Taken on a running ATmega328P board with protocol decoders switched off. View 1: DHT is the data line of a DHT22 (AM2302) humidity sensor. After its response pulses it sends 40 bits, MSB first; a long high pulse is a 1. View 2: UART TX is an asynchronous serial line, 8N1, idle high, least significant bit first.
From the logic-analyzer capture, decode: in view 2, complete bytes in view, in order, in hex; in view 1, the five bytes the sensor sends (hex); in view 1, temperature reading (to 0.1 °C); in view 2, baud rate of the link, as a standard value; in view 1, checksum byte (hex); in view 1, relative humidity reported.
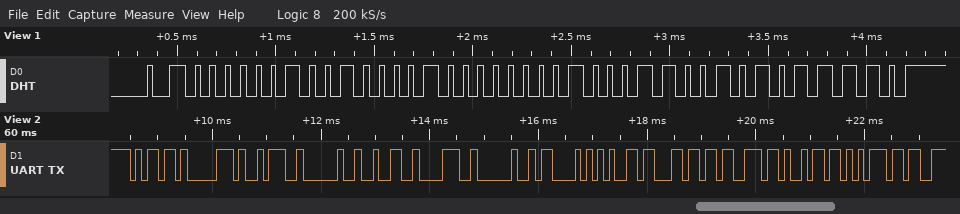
6D 70 3A 20 32 38 20 43 65 6C 73 69 75
02 42 01 19 5E
28.1 °C
9600 baud
0x5E
57.8 %
